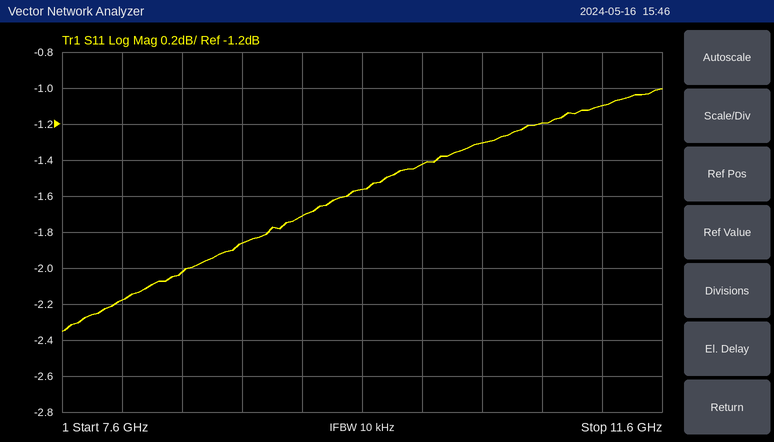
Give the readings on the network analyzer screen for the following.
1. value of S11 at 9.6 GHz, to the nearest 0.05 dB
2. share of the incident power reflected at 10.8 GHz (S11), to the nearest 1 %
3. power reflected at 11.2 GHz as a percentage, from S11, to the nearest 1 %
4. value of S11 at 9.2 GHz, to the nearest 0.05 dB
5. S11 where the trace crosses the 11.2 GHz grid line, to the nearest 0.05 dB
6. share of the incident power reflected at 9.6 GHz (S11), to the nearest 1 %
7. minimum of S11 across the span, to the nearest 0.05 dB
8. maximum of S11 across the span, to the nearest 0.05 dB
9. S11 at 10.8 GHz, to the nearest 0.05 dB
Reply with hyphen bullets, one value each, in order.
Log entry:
- -1.55 dB
- 76 %
- 78 %
- -1.70 dB
- -1.10 dB
- 70 %
- -2.35 dB
- -1.00 dB
- -1.20 dB
